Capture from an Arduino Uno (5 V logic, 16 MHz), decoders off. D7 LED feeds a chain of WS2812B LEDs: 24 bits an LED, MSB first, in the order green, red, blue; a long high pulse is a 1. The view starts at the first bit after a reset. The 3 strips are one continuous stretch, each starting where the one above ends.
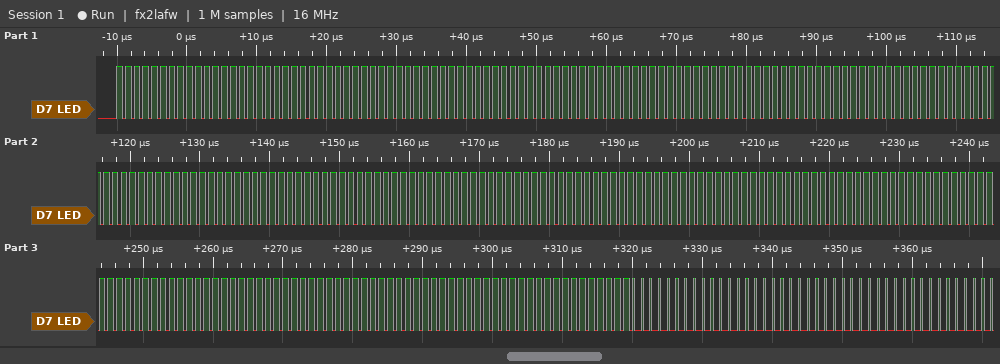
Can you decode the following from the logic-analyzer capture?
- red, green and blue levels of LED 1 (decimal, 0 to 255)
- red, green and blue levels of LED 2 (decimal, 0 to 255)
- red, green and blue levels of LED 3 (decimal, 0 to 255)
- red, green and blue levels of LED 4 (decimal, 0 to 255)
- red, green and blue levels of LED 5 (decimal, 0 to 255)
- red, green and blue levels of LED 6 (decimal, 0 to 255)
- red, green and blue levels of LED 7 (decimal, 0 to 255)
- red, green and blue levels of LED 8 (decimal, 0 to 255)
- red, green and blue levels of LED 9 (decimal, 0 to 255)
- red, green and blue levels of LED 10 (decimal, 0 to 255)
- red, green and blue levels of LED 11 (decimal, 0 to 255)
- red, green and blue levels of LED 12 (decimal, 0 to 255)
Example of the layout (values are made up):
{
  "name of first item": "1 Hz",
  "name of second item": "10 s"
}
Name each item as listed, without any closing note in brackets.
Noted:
{
  "red, green and blue levels of LED 1": "255, 255, 255",
  "red, green and blue levels of LED 2": "255, 255, 255",
  "red, green and blue levels of LED 3": "255, 255, 255",
  "red, green and blue levels of LED 4": "255, 255, 255",
  "red, green and blue levels of LED 5": "255, 255, 255",
  "red, green and blue levels of LED 6": "255, 255, 255",
  "red, green and blue levels of LED 7": "255, 255, 255",
  "red, green and blue levels of LED 8": "255, 255, 255",
  "red, green and blue levels of LED 9": "255, 255, 255",
  "red, green and blue levels of LED 10": "255, 255, 255",
  "red, green and blue levels of LED 11": "255, 255, 255",
  "red, green and blue levels of LED 12": "0, 0, 0"
}
